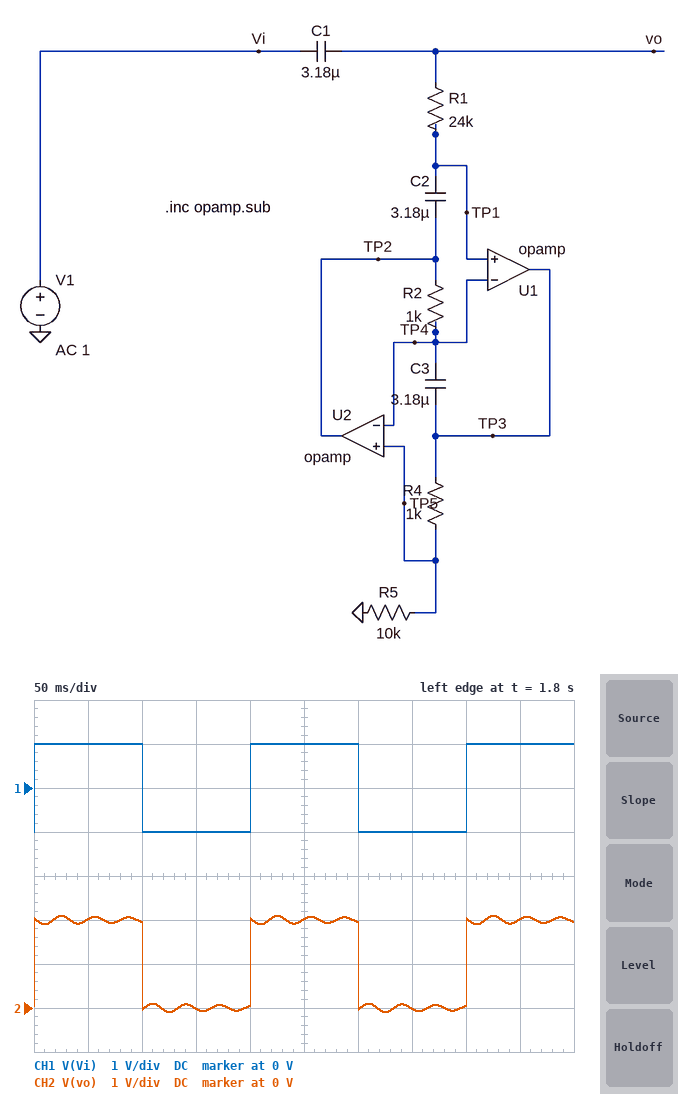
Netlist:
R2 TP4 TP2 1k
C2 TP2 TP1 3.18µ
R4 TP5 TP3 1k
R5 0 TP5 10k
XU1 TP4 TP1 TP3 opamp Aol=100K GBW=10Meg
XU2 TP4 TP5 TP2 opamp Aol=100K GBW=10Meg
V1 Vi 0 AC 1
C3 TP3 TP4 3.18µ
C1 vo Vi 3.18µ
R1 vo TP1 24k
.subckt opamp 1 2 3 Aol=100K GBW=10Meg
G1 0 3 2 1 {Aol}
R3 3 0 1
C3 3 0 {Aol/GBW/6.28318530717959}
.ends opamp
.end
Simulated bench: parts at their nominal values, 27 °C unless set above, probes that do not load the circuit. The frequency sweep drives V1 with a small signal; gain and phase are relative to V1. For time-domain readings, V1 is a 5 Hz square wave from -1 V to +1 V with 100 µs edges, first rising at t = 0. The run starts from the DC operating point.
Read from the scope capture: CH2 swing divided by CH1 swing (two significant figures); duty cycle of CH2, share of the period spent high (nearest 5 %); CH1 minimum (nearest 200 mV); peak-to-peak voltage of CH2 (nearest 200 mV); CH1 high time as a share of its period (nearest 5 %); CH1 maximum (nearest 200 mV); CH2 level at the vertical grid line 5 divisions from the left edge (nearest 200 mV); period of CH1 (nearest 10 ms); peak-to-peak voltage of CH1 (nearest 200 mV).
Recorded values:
1.1
50 %
-1.0 V
2.2 V
50 %
1.0 V
2.0 V
200 ms
2.0 V
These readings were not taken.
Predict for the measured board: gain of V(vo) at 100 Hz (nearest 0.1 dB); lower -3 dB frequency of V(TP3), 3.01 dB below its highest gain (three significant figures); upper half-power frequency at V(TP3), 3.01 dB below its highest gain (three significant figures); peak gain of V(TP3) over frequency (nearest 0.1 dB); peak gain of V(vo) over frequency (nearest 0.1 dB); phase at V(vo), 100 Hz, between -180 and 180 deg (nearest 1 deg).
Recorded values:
0 dB
31.2 Hz
33.3 Hz
24.6 dB
0 dB
1 deg
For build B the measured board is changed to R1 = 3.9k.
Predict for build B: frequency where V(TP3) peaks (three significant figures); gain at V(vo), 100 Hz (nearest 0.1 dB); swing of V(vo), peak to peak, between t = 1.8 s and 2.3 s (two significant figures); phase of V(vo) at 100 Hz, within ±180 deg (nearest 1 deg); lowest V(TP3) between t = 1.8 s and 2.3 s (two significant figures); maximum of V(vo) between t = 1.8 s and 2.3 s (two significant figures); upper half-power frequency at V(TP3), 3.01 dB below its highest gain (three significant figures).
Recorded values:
79.6 Hz
-0.5 dB
2.4 V
20 deg
-1.7 V
2.2 V
85.8 Hz
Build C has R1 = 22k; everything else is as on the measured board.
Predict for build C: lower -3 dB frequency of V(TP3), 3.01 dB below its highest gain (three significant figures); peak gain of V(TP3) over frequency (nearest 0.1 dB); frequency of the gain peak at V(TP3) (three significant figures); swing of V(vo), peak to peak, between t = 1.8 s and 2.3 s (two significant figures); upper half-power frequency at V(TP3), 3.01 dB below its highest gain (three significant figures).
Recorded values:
32.5 Hz
24.2 dB
33.7 Hz
2.3 V
34.8 Hz
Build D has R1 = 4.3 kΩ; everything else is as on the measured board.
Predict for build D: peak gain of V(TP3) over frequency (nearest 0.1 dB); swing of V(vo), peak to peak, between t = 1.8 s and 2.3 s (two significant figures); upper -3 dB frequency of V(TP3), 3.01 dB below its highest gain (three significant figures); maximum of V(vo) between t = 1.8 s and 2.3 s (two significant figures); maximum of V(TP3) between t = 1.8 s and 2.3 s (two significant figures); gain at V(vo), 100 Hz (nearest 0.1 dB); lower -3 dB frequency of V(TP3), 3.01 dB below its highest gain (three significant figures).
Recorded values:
17.2 dB
2.4 V
81.5 Hz
2.2 V
4.0 V
-0.3 dB
69.8 Hz
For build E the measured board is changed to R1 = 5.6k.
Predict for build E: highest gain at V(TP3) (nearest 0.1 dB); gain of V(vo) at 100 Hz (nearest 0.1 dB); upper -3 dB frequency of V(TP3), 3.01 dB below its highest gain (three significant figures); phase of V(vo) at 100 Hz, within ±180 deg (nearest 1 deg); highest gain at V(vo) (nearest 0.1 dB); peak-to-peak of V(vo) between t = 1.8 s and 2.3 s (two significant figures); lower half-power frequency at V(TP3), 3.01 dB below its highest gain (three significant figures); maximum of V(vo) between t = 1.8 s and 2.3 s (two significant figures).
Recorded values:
18.3 dB
-0.1 dB
70.9 Hz
9 deg
0 dB
2.4 V
61.9 Hz
2.2 V
